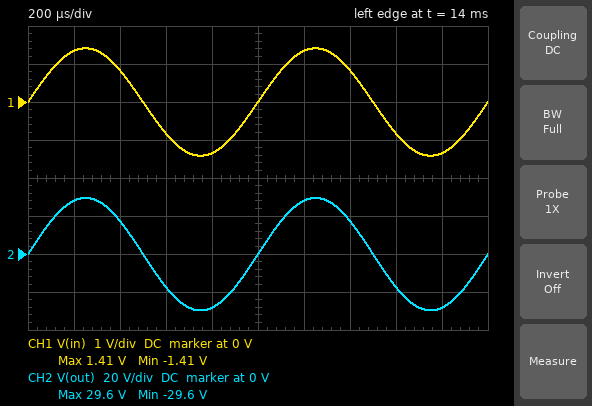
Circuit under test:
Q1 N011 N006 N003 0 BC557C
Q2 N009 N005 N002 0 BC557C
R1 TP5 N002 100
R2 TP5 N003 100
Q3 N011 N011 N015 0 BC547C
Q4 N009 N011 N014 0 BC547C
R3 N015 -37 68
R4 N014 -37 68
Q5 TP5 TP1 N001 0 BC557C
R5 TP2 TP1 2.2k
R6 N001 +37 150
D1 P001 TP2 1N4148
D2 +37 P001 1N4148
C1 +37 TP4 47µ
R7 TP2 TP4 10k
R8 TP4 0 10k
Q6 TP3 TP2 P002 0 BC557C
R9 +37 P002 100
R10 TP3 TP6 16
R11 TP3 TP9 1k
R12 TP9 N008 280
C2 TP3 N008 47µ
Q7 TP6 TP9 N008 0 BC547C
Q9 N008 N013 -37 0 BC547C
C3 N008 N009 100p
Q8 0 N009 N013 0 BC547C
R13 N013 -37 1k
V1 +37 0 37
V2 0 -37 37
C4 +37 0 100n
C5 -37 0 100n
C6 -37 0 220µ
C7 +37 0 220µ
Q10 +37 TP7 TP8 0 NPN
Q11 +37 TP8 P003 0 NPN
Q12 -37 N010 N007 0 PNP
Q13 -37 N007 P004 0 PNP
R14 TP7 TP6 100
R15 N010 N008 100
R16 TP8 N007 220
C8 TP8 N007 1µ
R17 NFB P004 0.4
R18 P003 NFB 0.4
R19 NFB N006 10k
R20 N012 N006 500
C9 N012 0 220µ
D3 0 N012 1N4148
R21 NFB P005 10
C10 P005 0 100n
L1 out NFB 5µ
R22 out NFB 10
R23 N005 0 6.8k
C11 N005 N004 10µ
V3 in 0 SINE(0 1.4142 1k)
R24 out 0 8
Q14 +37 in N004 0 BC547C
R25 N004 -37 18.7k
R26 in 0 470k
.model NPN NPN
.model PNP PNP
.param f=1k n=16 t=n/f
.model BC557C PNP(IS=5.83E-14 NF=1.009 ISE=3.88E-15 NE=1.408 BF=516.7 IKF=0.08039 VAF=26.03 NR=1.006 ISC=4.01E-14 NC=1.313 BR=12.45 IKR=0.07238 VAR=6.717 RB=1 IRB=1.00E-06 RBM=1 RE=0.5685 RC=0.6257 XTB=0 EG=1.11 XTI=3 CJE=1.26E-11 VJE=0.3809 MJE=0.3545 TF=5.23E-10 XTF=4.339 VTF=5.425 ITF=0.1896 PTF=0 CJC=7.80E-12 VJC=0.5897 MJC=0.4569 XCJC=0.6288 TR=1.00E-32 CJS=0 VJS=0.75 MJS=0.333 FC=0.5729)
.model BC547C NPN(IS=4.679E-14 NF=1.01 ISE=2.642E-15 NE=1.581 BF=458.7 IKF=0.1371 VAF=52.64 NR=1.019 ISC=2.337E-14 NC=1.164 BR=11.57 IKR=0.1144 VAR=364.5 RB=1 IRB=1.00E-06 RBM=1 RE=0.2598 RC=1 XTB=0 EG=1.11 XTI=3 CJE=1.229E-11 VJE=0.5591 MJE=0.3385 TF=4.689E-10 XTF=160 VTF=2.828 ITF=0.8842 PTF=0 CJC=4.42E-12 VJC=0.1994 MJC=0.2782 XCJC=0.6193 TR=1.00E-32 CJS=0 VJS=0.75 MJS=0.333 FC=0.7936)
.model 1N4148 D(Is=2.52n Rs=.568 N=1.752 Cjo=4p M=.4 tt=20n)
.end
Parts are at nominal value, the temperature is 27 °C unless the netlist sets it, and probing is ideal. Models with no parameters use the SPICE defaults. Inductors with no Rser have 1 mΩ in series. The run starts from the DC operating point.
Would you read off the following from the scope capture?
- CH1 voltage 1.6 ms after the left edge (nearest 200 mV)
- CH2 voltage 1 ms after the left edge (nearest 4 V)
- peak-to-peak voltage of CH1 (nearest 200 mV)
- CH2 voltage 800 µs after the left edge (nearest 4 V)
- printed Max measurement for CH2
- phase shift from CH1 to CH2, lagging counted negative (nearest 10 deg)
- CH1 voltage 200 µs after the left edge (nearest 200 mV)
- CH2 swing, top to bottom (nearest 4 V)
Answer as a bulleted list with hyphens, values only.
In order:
- -800 mV
- 0 V
- 2.8 V
- -28 V
- 29.6 V
- 0 deg
- 1.4 V
- 60 V
